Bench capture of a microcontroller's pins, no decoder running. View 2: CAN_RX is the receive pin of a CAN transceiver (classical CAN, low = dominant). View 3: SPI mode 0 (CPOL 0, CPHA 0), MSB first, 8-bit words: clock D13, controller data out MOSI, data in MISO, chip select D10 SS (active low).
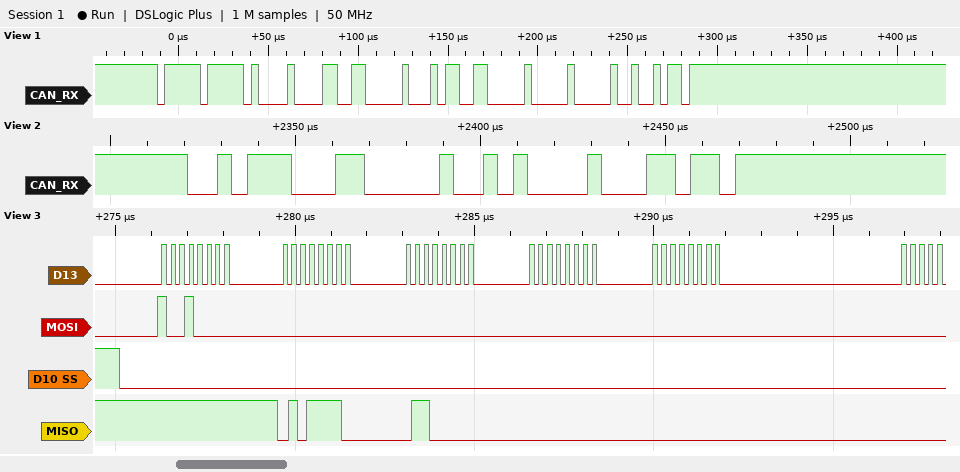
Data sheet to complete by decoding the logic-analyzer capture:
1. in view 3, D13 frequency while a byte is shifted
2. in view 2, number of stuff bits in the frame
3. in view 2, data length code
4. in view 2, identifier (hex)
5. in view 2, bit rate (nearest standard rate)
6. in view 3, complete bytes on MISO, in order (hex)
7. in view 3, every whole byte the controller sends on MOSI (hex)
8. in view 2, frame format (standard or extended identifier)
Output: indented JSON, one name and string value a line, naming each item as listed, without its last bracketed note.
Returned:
{
  "in view 3, D13 frequency while a byte is shifted": "4 MHz",
  "in view 2, number of stuff bits in the frame": "1",
  "in view 2, data length code": "0",
  "in view 2, identifier": "0x2E3",
  "in view 2, bit rate": "250 kbit/s",
  "in view 3, complete bytes on MISO, in order": "FF 5E 60 00 00",
  "in view 3, every whole byte the controller sends on MOSI": "90 00 00 00 00",
  "in view 2, frame format": "standard"
}
